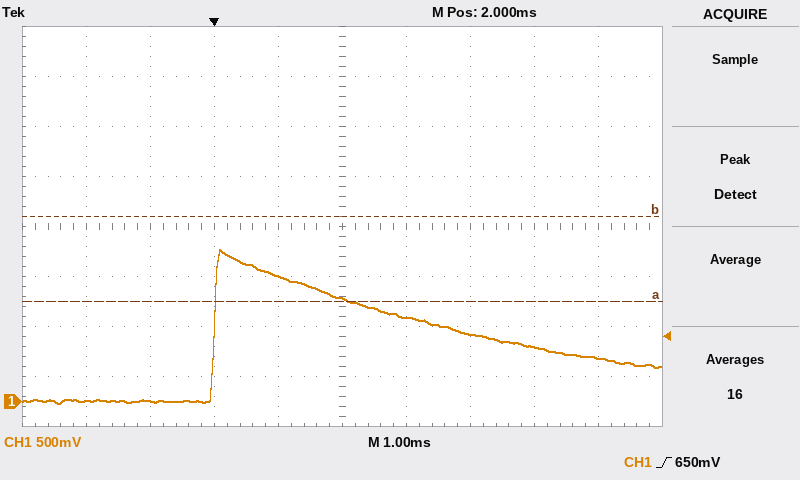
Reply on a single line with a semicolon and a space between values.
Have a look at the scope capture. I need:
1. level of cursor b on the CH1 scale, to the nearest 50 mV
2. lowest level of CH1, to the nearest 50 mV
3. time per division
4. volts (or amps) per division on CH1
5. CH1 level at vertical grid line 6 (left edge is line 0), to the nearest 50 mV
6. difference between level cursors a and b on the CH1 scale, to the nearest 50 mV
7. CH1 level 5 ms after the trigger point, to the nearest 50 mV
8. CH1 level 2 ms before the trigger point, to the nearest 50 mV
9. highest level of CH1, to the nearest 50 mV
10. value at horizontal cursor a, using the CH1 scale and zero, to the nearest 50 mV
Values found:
1.85 V; 0 mV; 1 ms; 500 mV; 850 mV; 850 mV; 550 mV; 0 mV; 1.50 V; 1.00 V
